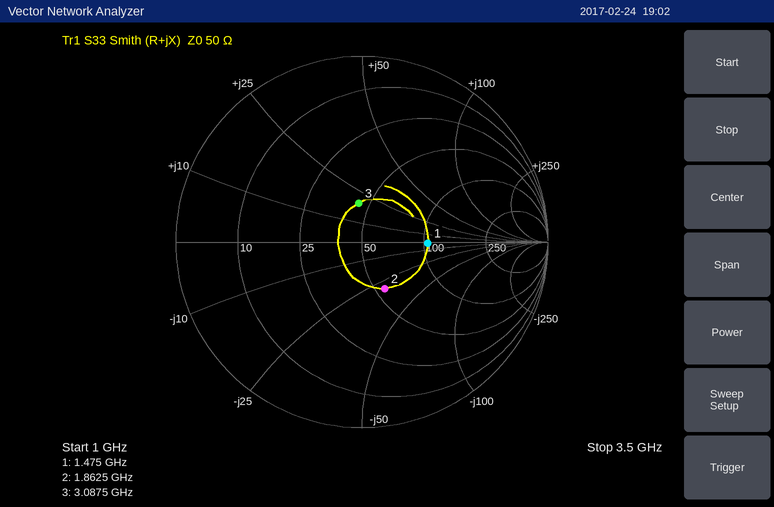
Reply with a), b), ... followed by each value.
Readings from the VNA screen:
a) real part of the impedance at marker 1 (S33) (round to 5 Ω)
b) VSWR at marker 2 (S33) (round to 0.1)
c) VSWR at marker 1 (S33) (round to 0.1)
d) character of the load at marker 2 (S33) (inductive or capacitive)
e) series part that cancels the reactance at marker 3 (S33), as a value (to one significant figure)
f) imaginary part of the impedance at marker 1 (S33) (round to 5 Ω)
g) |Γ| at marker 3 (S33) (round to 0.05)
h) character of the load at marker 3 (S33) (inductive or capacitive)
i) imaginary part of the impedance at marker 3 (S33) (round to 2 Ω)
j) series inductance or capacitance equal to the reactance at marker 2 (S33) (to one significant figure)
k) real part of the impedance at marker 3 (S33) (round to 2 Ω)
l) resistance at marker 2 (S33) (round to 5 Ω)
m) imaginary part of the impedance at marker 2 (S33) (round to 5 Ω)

a) 105 Ω
b) 1.8
c) 2.1
d) capacitive
e) 3 pF
f) 0 Ω
g) 0.20
h) inductive
i) +20 Ω
j) 3 pF
k) 44 Ω
l) 55 Ω
m) -30 Ω
